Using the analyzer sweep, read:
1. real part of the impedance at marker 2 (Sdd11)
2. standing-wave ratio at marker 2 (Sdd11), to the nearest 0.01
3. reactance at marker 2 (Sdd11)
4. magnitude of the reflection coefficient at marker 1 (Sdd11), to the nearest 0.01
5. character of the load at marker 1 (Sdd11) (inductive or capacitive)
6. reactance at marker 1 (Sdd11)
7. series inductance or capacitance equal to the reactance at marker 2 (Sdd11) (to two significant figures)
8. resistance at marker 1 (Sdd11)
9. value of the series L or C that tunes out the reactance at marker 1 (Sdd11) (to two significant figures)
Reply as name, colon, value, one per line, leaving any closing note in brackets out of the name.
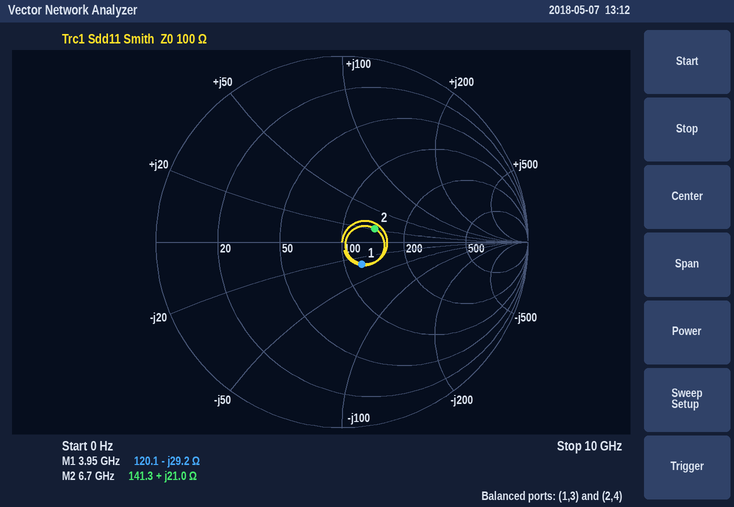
real part of the impedance at marker 2: 141.3 Ω
standing-wave ratio at marker 2 (Sdd11), to the nearest 0.01: 1.47
reactance at marker 2: +21.0 Ω
magnitude of the reflection coefficient at marker 1 (Sdd11), to the nearest 0.01: 0.16
character of the load at marker 1 (Sdd11): capacitive
reactance at marker 1: -29.2 Ω
series inductance or capacitance equal to the reactance at marker 2 (Sdd11): 500 pH
resistance at marker 1: 120.1 Ω
value of the series L or C that tunes out the reactance at marker 1 (Sdd11): 1.2 nH
